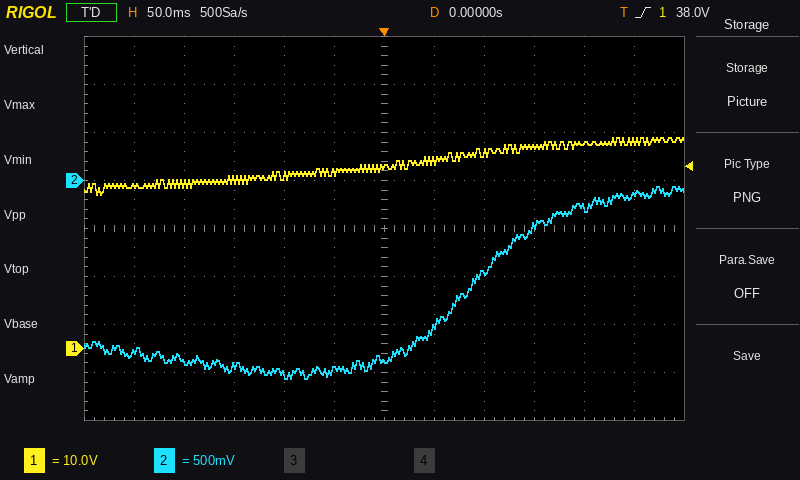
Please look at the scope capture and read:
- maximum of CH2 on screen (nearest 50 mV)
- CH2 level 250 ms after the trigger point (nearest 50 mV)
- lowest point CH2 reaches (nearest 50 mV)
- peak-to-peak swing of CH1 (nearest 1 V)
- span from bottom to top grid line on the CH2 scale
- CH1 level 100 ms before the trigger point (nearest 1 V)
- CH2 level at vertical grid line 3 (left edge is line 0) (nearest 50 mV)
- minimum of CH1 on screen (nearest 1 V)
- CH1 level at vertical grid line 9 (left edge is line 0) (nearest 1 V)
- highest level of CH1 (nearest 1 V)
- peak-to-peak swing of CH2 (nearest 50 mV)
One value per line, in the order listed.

-50 mV
-150 mV
-2.05 V
12 V
4 V
36 V
-1.95 V
32 V
42 V
44 V
2.00 V
